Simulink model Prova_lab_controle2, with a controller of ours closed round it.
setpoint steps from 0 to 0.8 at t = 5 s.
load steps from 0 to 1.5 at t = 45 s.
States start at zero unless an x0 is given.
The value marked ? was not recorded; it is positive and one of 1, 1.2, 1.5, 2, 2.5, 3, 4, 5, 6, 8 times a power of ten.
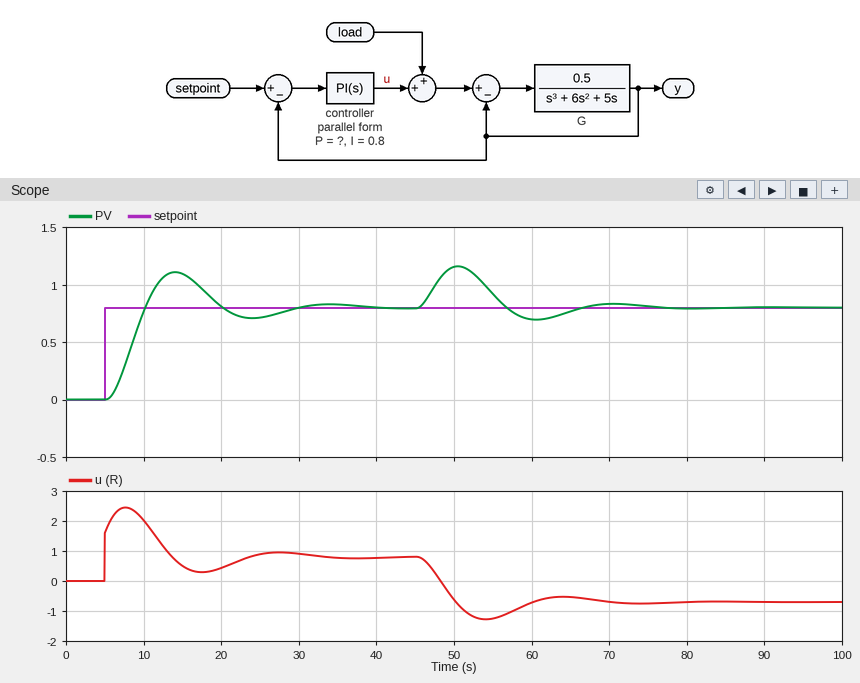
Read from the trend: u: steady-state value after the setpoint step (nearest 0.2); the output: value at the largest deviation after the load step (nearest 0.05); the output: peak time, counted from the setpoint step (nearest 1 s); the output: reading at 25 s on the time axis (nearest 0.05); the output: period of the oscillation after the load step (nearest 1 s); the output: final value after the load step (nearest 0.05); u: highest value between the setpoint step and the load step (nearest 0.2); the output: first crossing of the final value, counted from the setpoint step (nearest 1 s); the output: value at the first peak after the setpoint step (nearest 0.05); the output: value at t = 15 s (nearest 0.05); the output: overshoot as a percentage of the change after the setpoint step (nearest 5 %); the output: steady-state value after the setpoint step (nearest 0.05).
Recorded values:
0.8
1.15
9 s
0.70
20 s
0.80
2.4
5 s
1.10
1.10
40 %
0.80
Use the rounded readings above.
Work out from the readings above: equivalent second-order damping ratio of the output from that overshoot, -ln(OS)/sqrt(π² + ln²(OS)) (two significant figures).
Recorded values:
0.28
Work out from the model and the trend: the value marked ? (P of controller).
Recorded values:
2
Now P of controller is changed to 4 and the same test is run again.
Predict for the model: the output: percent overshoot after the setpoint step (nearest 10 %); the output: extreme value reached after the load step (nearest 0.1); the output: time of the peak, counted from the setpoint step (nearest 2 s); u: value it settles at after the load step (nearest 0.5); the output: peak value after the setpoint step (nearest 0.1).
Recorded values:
20 %
1.1
6 s
-0.5
1.0
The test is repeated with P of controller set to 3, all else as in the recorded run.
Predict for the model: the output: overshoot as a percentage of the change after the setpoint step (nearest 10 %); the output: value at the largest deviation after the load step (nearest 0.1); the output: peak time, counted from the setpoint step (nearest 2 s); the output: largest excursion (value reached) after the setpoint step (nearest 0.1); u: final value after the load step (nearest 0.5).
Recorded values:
30 %
1.1
8 s
1.0
-0.5
